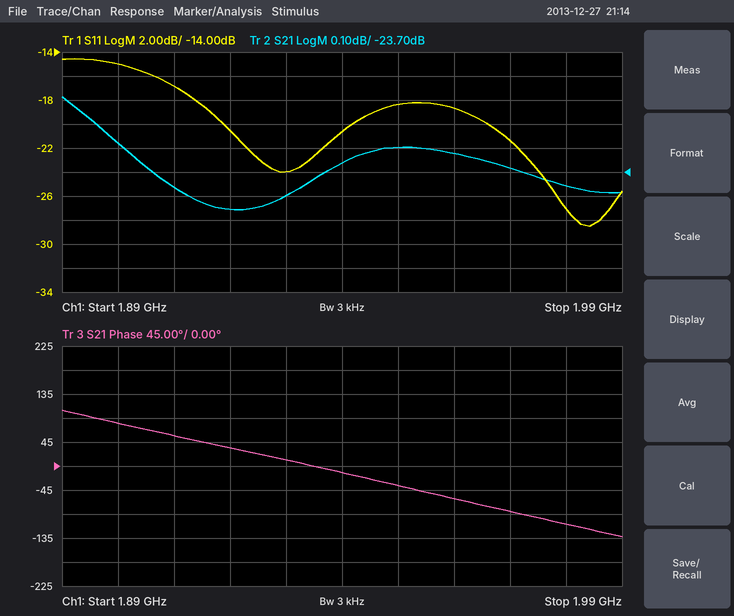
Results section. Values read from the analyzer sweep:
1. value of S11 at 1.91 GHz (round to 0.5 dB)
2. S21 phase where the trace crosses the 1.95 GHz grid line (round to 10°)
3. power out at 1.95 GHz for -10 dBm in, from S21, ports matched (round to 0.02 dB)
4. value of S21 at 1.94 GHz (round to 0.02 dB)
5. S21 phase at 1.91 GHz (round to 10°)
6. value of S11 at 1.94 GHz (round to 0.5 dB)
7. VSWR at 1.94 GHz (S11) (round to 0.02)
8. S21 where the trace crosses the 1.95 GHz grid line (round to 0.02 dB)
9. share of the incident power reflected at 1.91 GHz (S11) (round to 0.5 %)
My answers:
-17.0 dB
-40°
-33.60 dBm
-23.66 dB
60°
-20.5 dB
1.20
-23.60 dB
2.0 %
